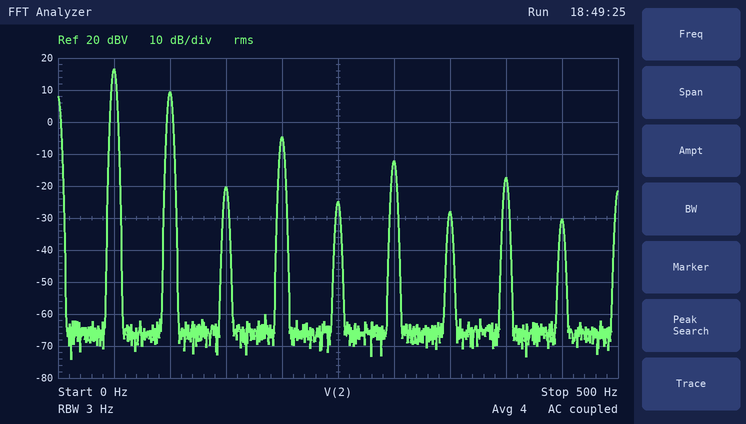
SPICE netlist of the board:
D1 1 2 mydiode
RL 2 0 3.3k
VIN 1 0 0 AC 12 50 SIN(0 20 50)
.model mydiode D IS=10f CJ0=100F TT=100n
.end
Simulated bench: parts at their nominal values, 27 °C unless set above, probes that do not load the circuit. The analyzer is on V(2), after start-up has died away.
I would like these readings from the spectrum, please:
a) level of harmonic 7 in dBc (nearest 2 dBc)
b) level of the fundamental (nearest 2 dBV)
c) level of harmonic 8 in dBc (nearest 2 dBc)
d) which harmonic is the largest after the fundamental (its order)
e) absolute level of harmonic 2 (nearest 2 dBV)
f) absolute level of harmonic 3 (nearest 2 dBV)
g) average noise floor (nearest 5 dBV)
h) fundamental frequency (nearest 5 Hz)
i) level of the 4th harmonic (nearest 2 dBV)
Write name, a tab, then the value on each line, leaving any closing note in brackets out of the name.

level of harmonic 7 in dBc	-44 dBc
level of the fundamental	16 dBV
level of harmonic 8 in dBc	-34 dBc
which harmonic is the largest after the fundamental	2
absolute level of harmonic 2	10 dBV
absolute level of harmonic 3	-20 dBV
average noise floor	-65 dBV
fundamental frequency	50 Hz
level of the 4th harmonic	-4 dBV
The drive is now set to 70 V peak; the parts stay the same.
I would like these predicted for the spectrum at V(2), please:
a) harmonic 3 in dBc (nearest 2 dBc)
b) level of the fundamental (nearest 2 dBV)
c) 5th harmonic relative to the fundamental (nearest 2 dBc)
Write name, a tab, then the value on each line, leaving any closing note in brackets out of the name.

harmonic 3 in dBc	-48 dBc
level of the fundamental	28 dBV
5th harmonic relative to the fundamental	-52 dBc
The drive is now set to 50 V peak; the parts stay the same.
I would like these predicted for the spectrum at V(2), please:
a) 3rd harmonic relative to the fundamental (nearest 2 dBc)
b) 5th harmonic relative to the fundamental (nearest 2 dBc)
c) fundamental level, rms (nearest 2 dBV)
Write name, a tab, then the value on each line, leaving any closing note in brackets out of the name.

3rd harmonic relative to the fundamental	-44 dBc
5th harmonic relative to the fundamental	-50 dBc
fundamental level, rms	24 dBV
